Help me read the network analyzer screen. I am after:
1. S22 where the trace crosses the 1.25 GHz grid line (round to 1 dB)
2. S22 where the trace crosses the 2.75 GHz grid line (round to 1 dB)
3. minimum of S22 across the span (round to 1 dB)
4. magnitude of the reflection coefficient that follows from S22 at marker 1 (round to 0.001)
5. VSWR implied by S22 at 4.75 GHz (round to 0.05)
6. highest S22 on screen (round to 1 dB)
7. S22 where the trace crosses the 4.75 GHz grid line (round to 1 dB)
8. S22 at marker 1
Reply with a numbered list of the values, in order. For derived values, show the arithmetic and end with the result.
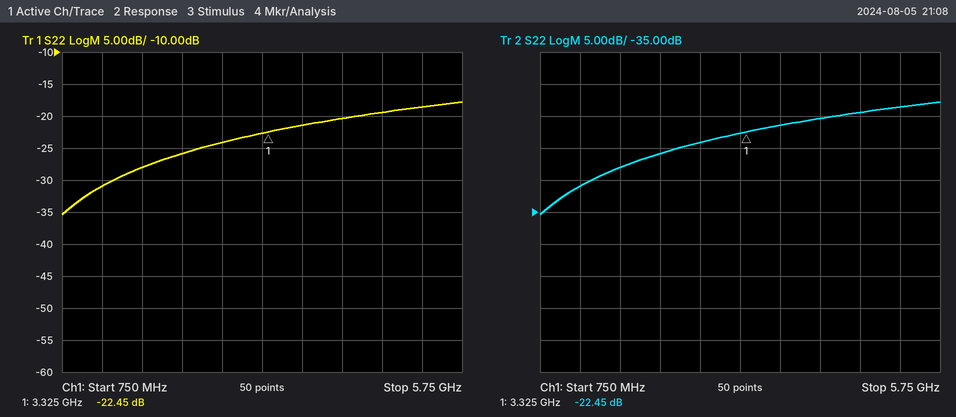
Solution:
1. -31 dB
2. -24 dB
3. -35 dB
4. 10^(-22.45/20) ≈ 0.075
5. |Γ| = 10^(-19/20) = 0.1122; VSWR = (1 + 0.1122)/(1 − 0.1122) ≈ 1.25
6. -18 dB
7. -19 dB
8. -22.45 dB
